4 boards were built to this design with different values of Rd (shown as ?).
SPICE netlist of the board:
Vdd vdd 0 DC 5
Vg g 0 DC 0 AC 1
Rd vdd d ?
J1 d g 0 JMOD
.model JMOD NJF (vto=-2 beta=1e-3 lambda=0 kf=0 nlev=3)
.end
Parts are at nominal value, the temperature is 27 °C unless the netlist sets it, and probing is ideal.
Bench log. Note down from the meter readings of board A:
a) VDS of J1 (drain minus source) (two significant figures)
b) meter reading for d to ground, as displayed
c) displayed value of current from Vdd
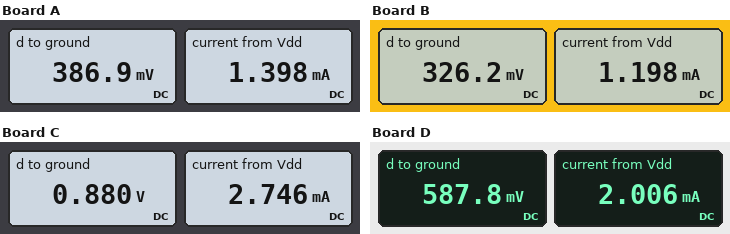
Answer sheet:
390 mV
386.9 mV
1.398 mA
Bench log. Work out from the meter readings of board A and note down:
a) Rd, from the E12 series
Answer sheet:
3.3 kΩ
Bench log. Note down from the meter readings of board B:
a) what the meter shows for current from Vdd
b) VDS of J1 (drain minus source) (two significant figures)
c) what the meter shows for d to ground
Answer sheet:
1.198 mA
330 mV
326.2 mV
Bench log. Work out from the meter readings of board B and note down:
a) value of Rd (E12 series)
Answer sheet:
3.9 kΩ
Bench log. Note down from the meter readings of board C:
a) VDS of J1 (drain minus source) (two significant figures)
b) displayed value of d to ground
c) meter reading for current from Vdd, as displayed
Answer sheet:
880 mV
0.880 V
2.746 mA
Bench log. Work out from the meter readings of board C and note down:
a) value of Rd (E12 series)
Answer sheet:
1.5 kΩ
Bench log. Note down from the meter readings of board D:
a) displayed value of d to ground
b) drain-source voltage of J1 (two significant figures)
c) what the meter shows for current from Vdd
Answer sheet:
587.8 mV
590 mV
2.006 mA
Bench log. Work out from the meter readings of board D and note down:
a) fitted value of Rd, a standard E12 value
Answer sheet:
2.2 kΩ
